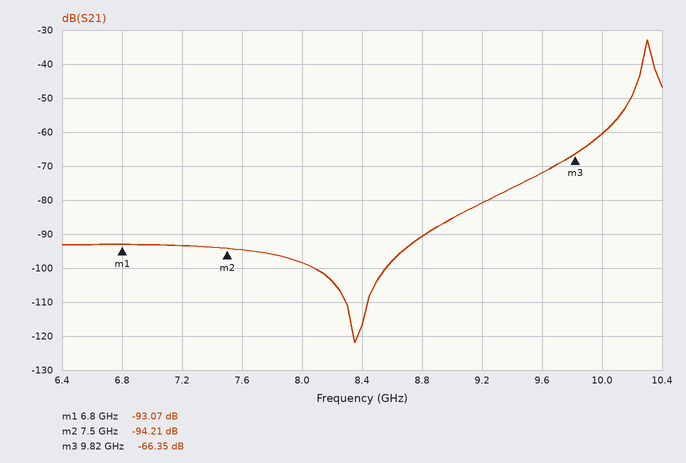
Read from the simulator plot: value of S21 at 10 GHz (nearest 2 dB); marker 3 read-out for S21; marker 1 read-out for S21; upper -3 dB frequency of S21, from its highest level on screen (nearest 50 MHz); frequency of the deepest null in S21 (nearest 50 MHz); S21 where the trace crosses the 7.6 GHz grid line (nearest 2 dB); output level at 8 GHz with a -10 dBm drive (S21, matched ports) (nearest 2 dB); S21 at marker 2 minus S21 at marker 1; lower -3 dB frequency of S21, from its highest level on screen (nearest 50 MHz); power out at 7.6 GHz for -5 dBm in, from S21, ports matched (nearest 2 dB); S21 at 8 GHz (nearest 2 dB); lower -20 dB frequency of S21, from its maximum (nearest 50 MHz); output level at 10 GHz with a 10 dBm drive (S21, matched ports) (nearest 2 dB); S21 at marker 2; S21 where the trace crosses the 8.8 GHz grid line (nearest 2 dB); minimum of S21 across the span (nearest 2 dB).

-60 dB
-66.35 dB
-93.07 dB
10.30 GHz
8.35 GHz
-94 dB
-108 dBm
-1.14 dB
10.30 GHz
-100 dBm
-98 dB
10.15 GHz
-50 dBm
-94.21 dB
-90 dB
-122 dB
